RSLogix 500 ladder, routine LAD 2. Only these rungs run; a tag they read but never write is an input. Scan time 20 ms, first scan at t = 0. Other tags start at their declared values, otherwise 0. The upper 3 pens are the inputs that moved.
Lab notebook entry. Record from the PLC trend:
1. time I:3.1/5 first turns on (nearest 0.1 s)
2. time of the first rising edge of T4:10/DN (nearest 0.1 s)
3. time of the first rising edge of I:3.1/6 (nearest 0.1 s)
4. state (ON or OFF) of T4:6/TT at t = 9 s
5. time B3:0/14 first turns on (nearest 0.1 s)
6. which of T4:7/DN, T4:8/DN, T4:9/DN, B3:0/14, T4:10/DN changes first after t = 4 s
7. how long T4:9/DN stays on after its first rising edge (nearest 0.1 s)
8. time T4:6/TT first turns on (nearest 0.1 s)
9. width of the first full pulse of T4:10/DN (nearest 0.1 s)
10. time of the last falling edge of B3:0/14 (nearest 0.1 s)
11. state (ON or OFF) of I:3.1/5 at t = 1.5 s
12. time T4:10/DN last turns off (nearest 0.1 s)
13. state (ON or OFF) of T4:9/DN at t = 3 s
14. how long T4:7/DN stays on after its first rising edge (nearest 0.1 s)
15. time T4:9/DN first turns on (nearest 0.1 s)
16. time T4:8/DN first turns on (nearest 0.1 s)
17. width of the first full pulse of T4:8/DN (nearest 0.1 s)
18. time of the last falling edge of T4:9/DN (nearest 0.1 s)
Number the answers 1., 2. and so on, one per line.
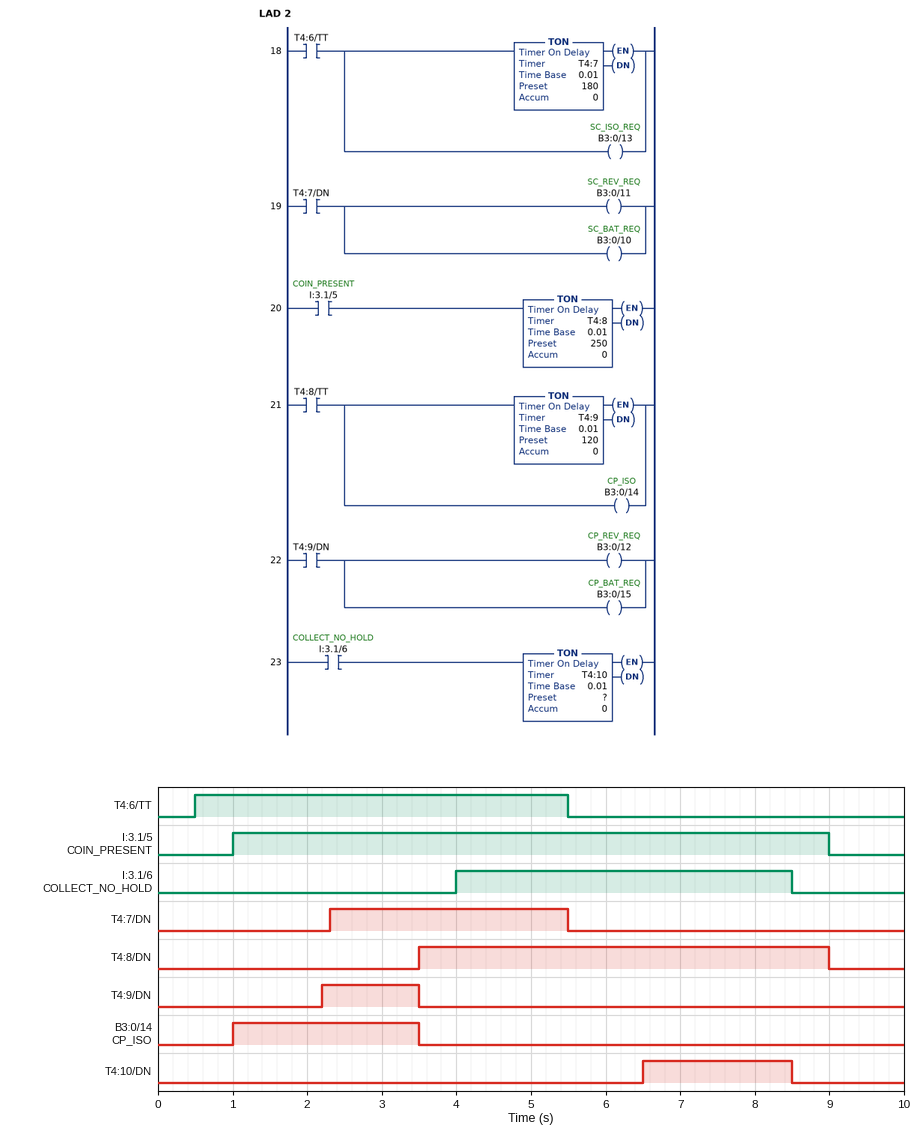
1. 1.0 s
2. 6.5 s
3. 4.0 s
4. OFF
5. 1.0 s
6. T4:7/DN
7. 1.3 s
8. 0.5 s
9. 2.0 s
10. 3.5 s
11. ON
12. 8.5 s
13. ON
14. 3.2 s
15. 2.2 s
16. 3.5 s
17. 5.5 s
18. 3.5 s
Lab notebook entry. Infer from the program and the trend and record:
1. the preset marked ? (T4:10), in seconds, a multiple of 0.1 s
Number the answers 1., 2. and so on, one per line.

1. 2.5 s
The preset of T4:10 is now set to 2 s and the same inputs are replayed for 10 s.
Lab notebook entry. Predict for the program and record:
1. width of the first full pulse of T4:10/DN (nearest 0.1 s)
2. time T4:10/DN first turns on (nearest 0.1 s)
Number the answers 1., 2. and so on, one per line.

1. 2.5 s
2. 6.0 s
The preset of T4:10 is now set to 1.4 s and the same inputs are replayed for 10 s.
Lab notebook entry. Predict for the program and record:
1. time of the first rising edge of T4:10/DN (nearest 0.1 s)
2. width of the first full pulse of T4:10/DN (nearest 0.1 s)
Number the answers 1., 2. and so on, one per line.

1. 5.4 s
2. 3.1 s
